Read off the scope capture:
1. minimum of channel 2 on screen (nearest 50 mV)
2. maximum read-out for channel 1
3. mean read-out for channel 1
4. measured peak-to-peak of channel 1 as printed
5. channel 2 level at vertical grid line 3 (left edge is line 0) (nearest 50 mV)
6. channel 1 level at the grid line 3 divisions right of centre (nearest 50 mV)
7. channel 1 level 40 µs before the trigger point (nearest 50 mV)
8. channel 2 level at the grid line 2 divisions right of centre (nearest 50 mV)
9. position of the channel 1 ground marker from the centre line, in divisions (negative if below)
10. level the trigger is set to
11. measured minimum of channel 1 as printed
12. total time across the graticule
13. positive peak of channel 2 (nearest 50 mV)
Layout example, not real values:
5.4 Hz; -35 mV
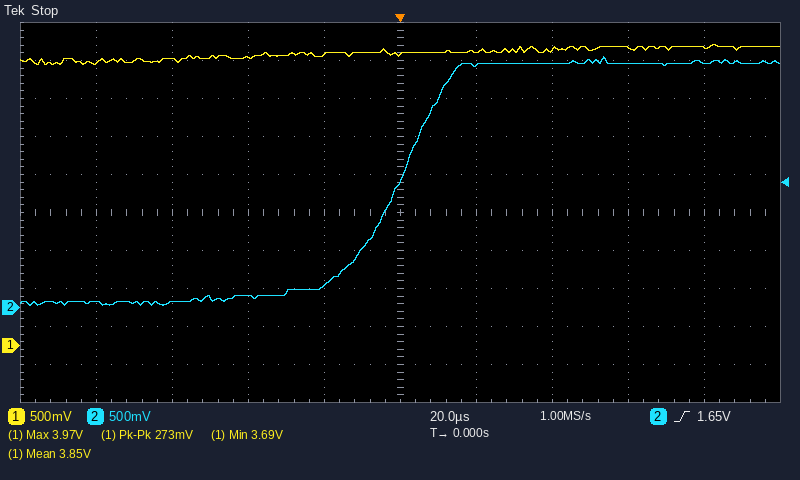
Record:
50 mV; 3.97 V; 3.85 V; 273 mV; 150 mV; 3.90 V; 3.80 V; 3.20 V; -3.5 div; 1.65 V; 3.69 V; 200 µs; 3.30 V
